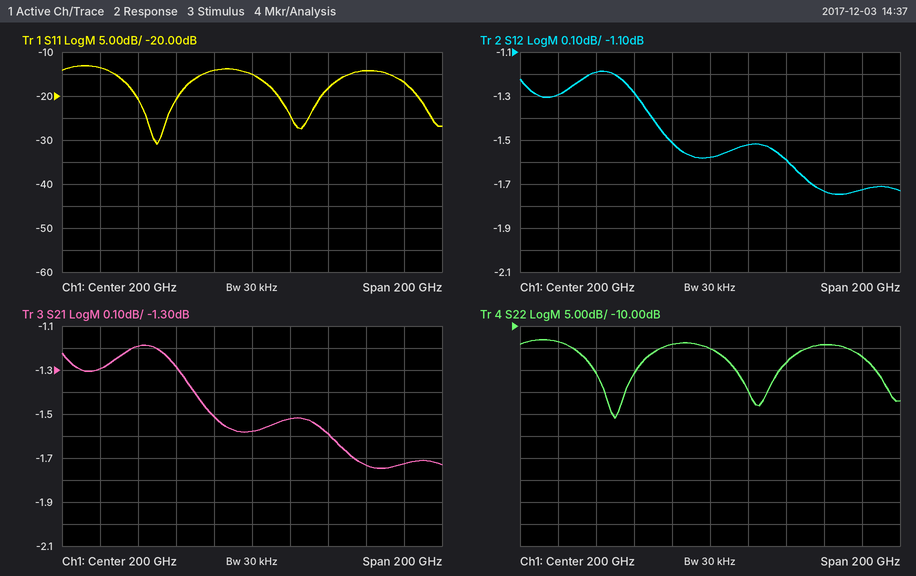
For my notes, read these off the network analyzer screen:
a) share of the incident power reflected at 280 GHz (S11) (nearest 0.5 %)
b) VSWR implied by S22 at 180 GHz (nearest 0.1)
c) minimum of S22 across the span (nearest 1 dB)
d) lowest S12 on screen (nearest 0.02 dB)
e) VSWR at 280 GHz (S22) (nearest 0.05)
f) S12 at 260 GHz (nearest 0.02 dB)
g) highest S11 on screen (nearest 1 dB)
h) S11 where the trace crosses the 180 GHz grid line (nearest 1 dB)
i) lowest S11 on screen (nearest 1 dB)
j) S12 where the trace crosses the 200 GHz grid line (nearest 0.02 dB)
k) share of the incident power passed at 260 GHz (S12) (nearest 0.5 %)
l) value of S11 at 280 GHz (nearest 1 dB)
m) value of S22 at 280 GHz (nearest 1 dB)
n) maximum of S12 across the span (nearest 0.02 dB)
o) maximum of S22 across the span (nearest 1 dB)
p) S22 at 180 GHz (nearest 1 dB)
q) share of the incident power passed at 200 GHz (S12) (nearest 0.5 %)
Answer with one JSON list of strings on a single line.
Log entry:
["2.0 %", "1.5", "-31 dB", "-1.74 dB", "1.35", "-1.74 dB", "-13 dB", "-14 dB", "-31 dB", "-1.58 dB", "67.0 %", "-17 dB", "-17 dB", "-1.18 dB", "-13 dB", "-14 dB", "69.5 %"]
